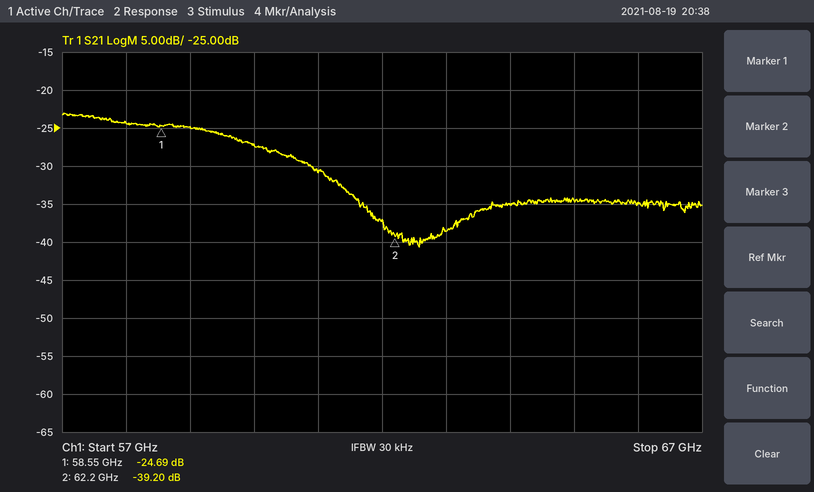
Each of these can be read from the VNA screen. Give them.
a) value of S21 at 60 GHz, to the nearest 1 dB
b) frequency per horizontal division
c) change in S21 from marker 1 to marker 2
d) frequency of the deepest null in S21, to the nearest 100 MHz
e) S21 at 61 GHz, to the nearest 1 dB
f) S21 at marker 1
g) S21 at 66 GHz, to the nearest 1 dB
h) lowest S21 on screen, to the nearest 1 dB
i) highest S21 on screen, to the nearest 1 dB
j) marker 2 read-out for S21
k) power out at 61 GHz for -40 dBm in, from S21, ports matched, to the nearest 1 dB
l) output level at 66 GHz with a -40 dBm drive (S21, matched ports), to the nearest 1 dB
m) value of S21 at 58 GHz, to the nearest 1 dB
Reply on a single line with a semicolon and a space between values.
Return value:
-27 dB; 1 GHz; -14.51 dB; 62.6 GHz; -31 dB; -24.69 dB; -35 dB; -41 dB; -23 dB; -39.20 dB; -71 dBm; -75 dBm; -24 dB
